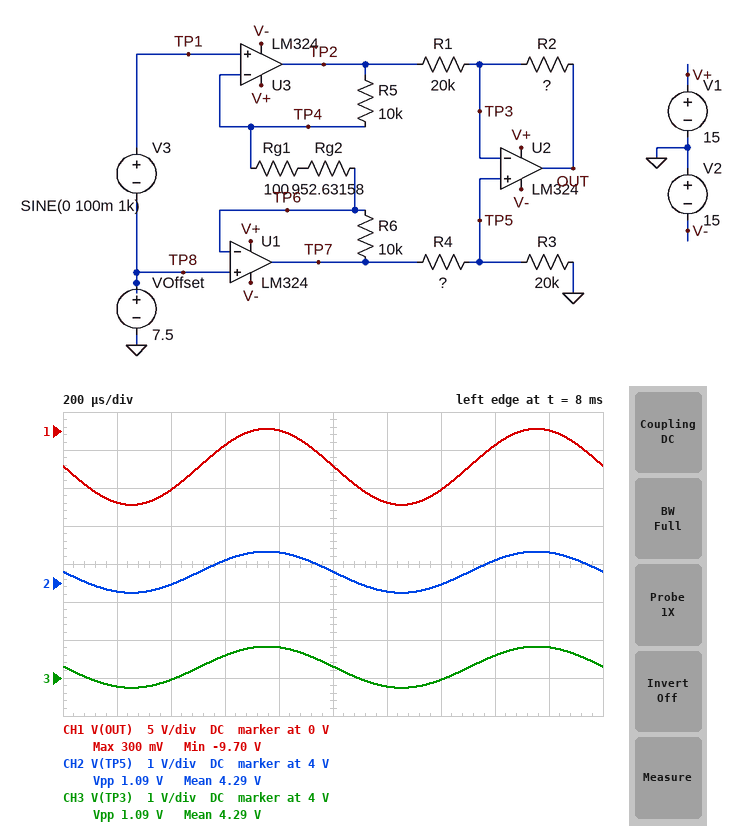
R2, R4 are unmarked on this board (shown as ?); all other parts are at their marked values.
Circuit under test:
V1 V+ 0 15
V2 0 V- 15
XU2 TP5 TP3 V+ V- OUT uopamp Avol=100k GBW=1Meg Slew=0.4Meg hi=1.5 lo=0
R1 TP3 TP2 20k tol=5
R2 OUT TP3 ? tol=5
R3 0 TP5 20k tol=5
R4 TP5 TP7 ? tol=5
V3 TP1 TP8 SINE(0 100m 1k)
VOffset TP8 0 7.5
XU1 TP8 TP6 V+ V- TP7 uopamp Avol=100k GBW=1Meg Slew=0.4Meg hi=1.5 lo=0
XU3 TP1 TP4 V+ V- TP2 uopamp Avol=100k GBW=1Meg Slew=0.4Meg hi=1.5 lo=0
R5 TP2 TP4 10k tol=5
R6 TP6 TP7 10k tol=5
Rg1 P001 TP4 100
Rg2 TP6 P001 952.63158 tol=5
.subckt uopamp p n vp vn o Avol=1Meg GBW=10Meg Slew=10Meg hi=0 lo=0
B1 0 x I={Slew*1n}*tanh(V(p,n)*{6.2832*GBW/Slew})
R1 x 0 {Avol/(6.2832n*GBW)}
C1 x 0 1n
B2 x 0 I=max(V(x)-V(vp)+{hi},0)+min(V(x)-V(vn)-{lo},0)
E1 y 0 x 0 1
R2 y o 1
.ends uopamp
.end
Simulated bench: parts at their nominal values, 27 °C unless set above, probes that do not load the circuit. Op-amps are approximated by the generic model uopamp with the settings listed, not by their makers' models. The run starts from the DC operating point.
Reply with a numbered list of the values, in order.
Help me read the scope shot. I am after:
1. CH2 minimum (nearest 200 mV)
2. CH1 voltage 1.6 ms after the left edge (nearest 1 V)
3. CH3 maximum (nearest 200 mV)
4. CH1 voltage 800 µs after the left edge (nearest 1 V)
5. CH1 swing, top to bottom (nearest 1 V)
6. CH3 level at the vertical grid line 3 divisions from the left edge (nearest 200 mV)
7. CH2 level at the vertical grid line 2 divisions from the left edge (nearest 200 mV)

1. 3.8 V
2. -2 V
3. 4.8 V
4. 0 V
5. 10 V
6. 4.6 V
7. 4.0 V
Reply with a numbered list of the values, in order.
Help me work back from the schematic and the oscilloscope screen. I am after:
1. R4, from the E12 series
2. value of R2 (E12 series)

1. 15 kΩ
2. 56 kΩ
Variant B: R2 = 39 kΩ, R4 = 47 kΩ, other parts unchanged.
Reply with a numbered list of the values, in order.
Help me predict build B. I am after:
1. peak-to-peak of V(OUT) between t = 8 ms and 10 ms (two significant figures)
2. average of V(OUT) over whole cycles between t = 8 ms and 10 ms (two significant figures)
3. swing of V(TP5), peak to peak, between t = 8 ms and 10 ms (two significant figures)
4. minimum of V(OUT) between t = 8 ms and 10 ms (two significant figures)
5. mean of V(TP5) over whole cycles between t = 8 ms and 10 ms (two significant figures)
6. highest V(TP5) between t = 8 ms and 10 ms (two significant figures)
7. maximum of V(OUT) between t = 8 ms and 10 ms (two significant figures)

1. 5.8 V
2. -8.0 V
3. 570 mV
4. -11 V
5. 2.2 V
6. 2.5 V
7. -5.1 V
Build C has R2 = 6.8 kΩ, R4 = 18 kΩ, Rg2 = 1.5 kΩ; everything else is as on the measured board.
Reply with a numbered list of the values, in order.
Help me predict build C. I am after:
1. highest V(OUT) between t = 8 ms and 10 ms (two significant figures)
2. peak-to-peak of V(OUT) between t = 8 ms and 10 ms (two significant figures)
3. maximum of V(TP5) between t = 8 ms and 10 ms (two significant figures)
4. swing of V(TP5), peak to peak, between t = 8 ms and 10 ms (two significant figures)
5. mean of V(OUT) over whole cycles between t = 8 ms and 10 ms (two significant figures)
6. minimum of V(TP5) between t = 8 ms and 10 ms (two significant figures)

1. 3.4 V
2. 1.4 V
3. 4.3 V
4. 660 mV
5. 2.7 V
6. 3.6 V
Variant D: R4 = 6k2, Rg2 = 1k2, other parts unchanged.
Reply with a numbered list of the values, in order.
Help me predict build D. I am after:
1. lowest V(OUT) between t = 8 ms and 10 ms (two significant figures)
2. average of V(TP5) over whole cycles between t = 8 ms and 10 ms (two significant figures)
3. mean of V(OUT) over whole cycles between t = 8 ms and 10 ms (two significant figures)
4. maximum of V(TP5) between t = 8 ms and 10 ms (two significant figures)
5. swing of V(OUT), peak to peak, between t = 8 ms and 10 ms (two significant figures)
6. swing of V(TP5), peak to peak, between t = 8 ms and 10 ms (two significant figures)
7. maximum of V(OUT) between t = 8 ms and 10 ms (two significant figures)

1. -3.9 V
2. 5.7 V
3. 760 mV
4. 6.3 V
5. 9.3 V
6. 1.2 V
7. 5.4 V
